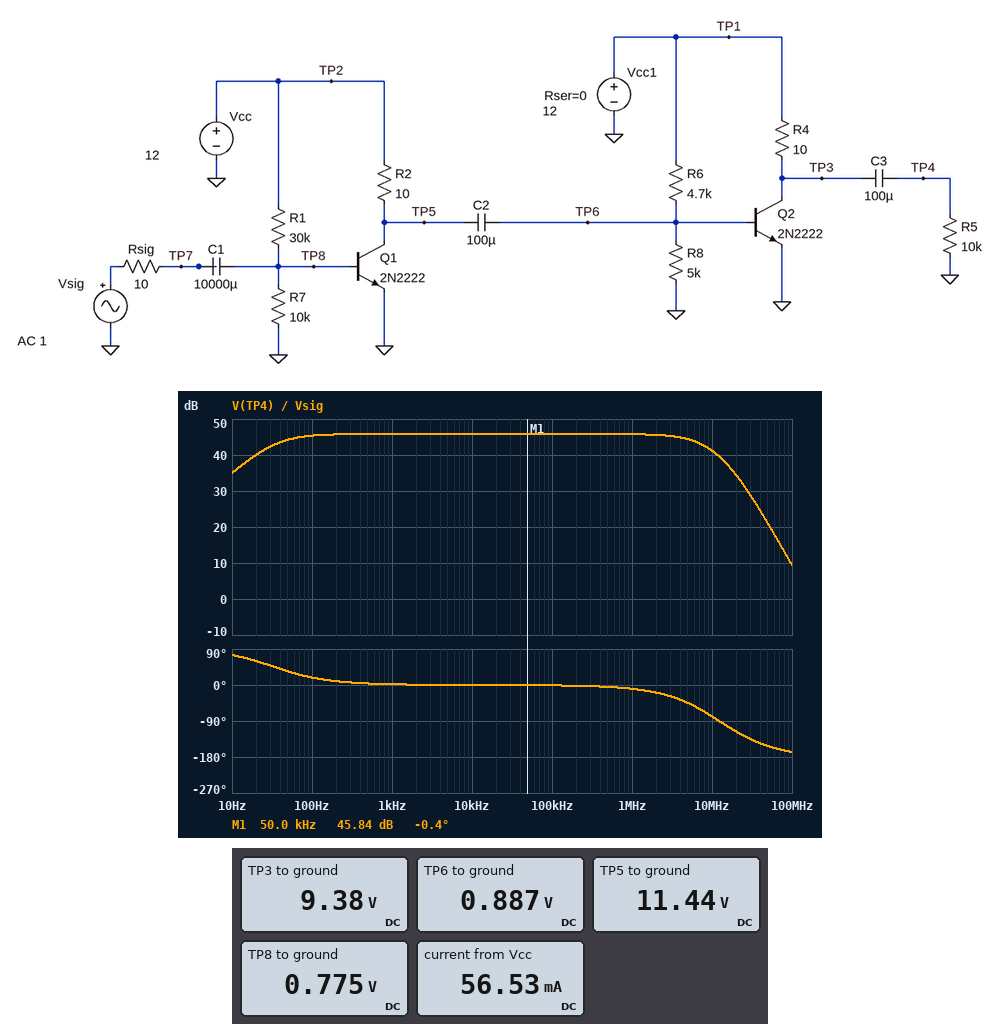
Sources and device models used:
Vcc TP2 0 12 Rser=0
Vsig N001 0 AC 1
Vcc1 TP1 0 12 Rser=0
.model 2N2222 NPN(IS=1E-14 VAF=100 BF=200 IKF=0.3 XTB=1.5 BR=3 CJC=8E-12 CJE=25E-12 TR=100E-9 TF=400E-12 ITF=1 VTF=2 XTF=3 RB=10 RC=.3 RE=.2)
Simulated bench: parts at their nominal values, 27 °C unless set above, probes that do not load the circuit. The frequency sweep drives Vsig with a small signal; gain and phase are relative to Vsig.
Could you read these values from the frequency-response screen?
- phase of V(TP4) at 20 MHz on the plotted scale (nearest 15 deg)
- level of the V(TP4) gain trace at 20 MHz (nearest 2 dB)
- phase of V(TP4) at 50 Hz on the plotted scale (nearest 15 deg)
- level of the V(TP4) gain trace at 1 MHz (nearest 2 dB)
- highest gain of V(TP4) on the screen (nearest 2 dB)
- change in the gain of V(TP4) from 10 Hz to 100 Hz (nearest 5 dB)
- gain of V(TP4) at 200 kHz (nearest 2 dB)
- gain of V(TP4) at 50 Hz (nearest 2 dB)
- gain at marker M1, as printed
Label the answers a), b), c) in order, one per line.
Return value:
a) -120 deg
b) 34 dB
c) 30 deg
d) 46 dB
e) 46 dB
f) 10 dB
g) 46 dB
h) 44 dB
i) 45.84 dB
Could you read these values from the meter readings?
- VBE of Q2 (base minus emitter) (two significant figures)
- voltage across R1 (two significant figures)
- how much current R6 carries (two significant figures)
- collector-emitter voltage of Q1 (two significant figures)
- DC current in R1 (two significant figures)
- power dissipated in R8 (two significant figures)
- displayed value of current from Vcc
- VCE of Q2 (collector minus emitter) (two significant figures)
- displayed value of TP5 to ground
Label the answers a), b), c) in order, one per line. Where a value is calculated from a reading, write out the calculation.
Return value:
a) 887 mV = 890 mV
b) 12 V - 775 mV = 11 V
c) (12 V - 887 mV) / 4.7 kΩ = 2.4 mA
d) 11.44 V = 11 V
e) (12 V - 775 mV) / 30 kΩ = 370 µA
f) (887 mV)^2 / 5 kΩ = 160 µW
g) 56.53 mA
h) 9.38 V = 9.4 V
i) 11.44 V
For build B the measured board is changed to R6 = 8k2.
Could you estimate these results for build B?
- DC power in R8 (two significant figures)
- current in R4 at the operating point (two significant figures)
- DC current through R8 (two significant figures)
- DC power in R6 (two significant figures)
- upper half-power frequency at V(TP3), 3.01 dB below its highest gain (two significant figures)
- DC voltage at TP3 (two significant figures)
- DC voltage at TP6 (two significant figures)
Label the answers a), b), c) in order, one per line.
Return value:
a) 140 µW
b) 170 mA
c) 170 µA
d) 15 mW
e) 7.8 MHz
f) 10 V
g) 840 mV
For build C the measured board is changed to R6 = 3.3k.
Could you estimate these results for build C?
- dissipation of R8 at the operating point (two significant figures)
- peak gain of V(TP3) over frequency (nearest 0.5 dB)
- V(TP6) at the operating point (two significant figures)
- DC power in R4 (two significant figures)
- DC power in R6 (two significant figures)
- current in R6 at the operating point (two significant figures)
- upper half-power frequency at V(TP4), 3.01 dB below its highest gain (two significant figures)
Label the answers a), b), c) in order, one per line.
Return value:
a) 170 µW
b) 45.5 dB
c) 920 mV
d) 1.1 W
e) 37 mW
f) 3.4 mA
g) 7.5 MHz
